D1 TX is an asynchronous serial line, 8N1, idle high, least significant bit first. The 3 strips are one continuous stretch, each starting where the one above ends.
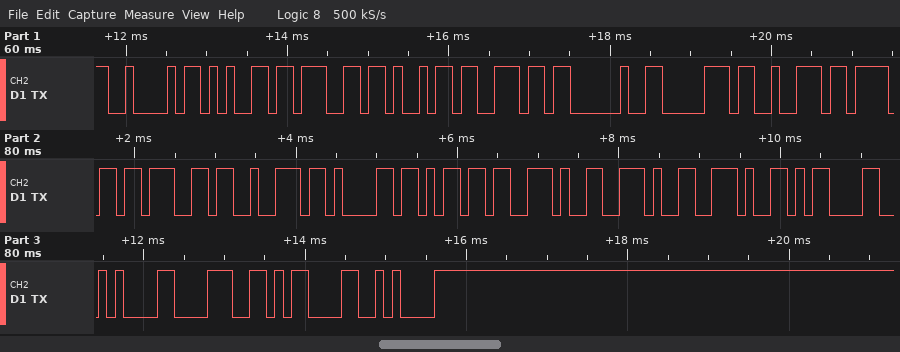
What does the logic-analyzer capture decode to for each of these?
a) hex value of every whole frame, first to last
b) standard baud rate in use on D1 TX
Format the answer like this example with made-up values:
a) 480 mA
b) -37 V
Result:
a) 42 65 67 69 6E 20 70 72 6F 67 72 61 6D 2E 2E 2E 0D 0A 38 0D 0A
b) 9600 baud
